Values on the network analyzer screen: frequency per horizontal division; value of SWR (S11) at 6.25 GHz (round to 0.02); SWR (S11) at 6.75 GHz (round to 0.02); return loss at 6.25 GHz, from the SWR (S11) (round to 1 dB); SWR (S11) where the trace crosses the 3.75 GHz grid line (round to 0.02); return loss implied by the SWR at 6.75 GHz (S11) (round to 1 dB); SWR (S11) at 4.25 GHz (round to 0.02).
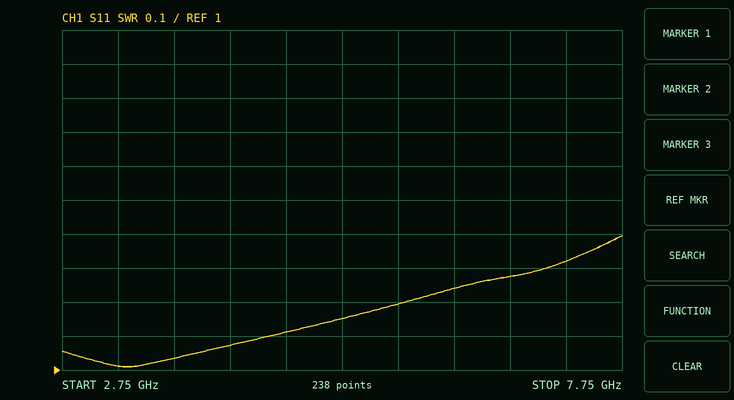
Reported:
500 MHz
1.24
1.28
19 dB
1.04
18 dB
1.08
